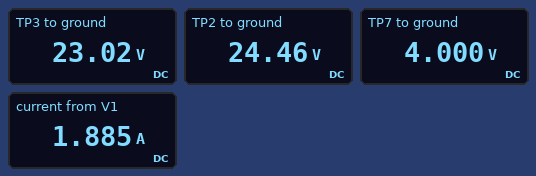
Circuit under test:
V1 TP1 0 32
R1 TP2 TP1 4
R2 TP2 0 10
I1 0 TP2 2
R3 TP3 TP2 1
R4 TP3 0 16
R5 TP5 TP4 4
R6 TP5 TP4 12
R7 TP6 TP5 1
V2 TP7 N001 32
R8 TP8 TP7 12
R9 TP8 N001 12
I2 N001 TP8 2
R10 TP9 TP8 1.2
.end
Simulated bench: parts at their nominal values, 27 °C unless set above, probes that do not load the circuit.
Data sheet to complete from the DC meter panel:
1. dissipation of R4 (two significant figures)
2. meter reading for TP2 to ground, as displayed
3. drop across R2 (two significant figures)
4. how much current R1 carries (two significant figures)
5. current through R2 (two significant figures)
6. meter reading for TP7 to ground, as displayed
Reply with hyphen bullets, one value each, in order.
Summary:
- 33 W
- 24.46 V
- 24 V
- 1.9 A
- 2.4 A
- 4.000 V
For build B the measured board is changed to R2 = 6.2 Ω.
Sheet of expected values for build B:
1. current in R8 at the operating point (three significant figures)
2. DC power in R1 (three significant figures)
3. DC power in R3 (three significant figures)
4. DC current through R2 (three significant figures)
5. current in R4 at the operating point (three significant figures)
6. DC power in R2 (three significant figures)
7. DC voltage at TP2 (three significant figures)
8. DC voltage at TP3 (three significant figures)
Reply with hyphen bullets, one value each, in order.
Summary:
- 333 mA
- 28.8 W
- 1.57 W
- 3.43 A
- 1.25 A
- 73.0 W
- 21.3 V
- 20.0 V
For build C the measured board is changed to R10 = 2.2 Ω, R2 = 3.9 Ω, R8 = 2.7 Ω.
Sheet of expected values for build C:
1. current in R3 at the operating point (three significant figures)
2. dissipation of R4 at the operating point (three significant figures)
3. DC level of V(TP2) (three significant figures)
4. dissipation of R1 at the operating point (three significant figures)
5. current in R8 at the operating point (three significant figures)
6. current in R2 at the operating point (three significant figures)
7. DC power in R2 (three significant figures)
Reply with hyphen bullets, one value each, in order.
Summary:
- 1.04 A
- 17.3 W
- 17.7 V
- 51.2 W
- 544 mA
- 4.54 A
- 80.3 W
